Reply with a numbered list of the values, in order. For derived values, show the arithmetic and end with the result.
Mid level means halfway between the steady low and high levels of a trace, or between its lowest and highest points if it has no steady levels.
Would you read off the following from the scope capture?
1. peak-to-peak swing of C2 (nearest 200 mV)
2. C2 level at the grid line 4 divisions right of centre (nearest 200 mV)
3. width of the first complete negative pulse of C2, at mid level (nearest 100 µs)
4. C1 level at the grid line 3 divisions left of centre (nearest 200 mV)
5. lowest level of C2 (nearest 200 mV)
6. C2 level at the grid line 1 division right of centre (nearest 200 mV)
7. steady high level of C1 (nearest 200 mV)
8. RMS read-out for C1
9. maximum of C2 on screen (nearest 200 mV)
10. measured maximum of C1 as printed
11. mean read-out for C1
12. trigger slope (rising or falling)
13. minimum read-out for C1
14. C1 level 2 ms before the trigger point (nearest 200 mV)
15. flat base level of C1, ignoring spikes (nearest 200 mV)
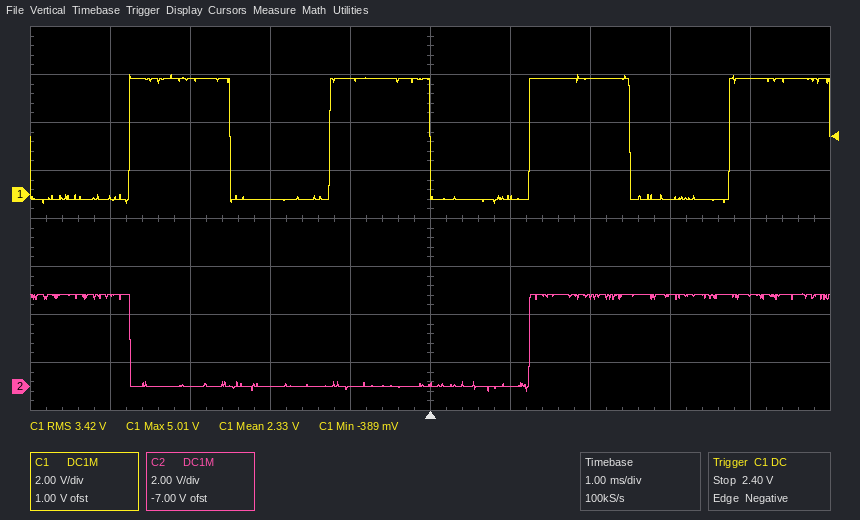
1. 3.8 V − (-200 mV) = 4.0 V
2. 3.8 V
3. 5.0 ms
4. 4.8 V
5. -200 mV
6. 0.0 V
7. 4.8 V
8. 3.42 V
9. 3.8 V
10. 5.01 V
11. 2.33 V
12. falling
13. -389 mV
14. -200 mV
15. -200 mV
